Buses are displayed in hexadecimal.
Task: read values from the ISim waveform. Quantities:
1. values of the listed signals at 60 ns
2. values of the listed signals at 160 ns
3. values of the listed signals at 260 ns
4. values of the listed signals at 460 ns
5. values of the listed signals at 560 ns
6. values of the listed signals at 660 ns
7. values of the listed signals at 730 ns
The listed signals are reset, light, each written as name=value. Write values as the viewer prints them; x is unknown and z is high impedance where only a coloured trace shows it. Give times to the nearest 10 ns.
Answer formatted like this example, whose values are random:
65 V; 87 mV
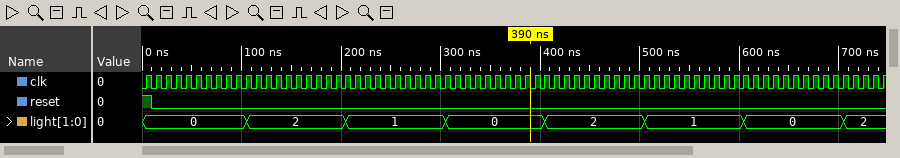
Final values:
reset=0, light=0; reset=0, light=2; reset=0, light=1; reset=0, light=2; reset=0, light=1; reset=0, light=0; reset=0, light=2
